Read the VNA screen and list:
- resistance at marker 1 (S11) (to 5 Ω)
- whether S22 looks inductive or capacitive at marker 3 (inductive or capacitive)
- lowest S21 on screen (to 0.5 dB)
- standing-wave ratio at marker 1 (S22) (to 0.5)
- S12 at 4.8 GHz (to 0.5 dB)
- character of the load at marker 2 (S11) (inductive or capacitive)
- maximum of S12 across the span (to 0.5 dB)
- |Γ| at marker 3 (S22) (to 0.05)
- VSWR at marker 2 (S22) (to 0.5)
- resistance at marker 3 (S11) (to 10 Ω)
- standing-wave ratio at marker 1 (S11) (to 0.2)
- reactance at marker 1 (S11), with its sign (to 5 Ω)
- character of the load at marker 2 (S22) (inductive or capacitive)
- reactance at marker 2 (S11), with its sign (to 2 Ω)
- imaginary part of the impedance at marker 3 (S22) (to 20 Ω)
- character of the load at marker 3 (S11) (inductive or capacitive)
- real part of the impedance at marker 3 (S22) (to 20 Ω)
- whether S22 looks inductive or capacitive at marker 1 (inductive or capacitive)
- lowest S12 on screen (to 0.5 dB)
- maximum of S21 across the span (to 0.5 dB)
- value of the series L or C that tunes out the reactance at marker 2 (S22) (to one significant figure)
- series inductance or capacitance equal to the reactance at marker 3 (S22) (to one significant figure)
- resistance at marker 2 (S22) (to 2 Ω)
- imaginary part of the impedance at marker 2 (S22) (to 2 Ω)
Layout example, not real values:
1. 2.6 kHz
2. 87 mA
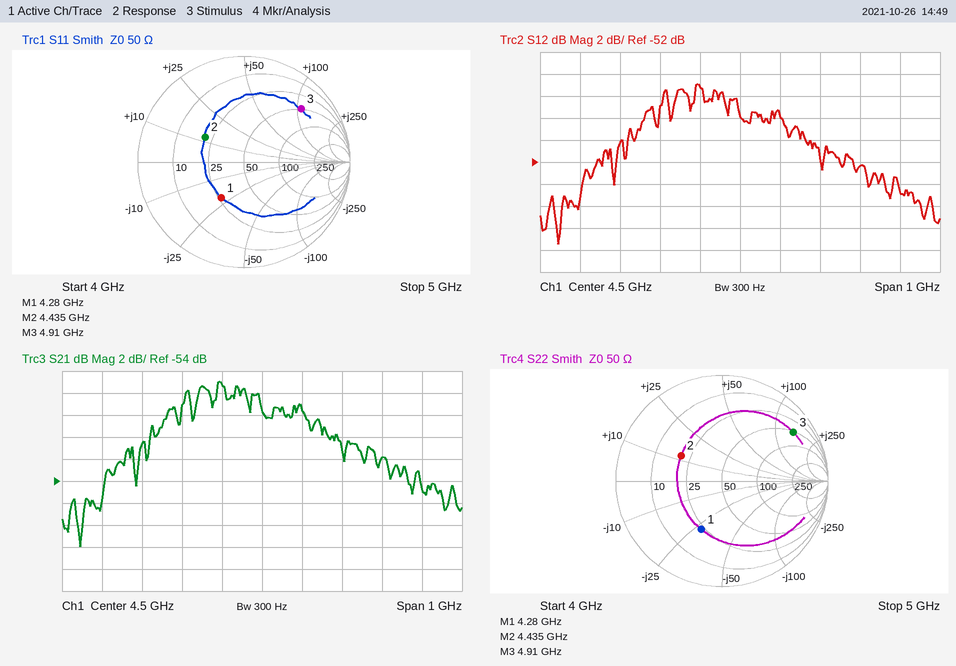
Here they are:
1. 25 Ω
2. inductive
3. -60.0 dB
4. 3.0
5. -52.5 dB
6. inductive
7. -45.0 dB
8. 0.80
9. 2.5
10. 50 Ω
11. 2.4
12. -20 Ω
13. inductive
14. +12 Ω
15. +140 Ω
16. inductive
17. 60 Ω
18. capacitive
19. -59.5 dB
20. -45.0 dB
21. 3 pF
22. 5 nH
23. 20 Ω
24. +12 Ω
